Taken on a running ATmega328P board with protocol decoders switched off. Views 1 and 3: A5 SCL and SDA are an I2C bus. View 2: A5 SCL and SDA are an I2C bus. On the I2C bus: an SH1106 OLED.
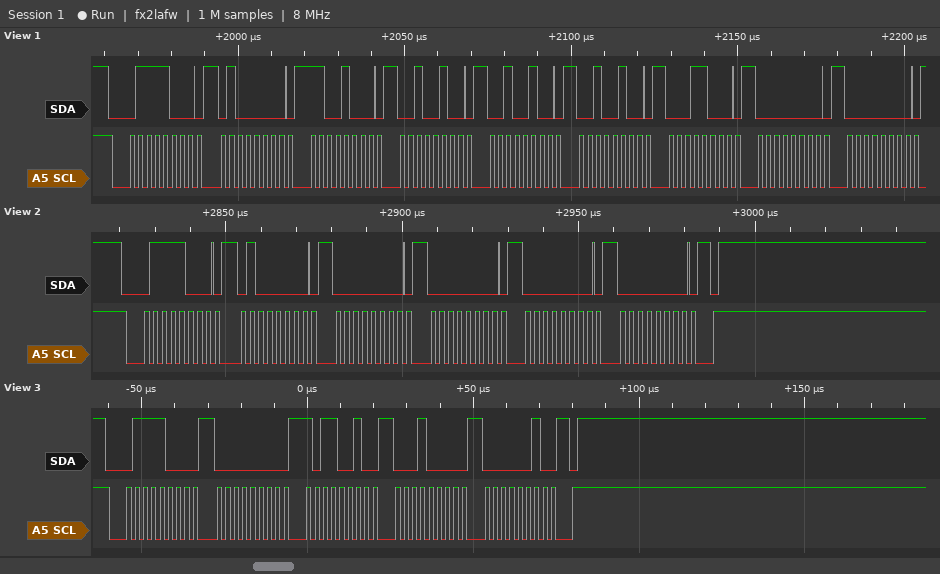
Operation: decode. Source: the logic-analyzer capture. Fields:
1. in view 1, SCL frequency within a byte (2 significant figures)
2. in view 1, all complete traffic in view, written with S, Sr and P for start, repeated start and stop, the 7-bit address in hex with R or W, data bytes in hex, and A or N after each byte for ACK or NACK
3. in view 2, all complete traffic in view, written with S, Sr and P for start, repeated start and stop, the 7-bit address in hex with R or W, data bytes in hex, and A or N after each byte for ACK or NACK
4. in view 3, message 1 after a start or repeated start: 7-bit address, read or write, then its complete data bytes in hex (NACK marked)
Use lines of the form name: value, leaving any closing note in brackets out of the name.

in view 1, SCL frequency within a byte: 400 kHz
in view 1, all complete traffic in view, written with S, Sr and P for start, repeated start and stop, the 7-bit address in hex with R or W, data bytes in hex, and A or N after each byte for ACK or NACK: S 3CW A 40 A C8 A 24 A 24 A 24 A 18 A 00 A 00 A
in view 2, all complete traffic in view, written with S, Sr and P for start, repeated start and stop, the 7-bit address in hex with R or W, data bytes in hex, and A or N after each byte for ACK or NACK: S 3CW A 40 A 00 A 00 A 00 A 00 A P
in view 3, message 1 after a start or repeated start: 7-bit address, read or write, then its complete data bytes in hex: 0x3C write: 00 B2 10 02
